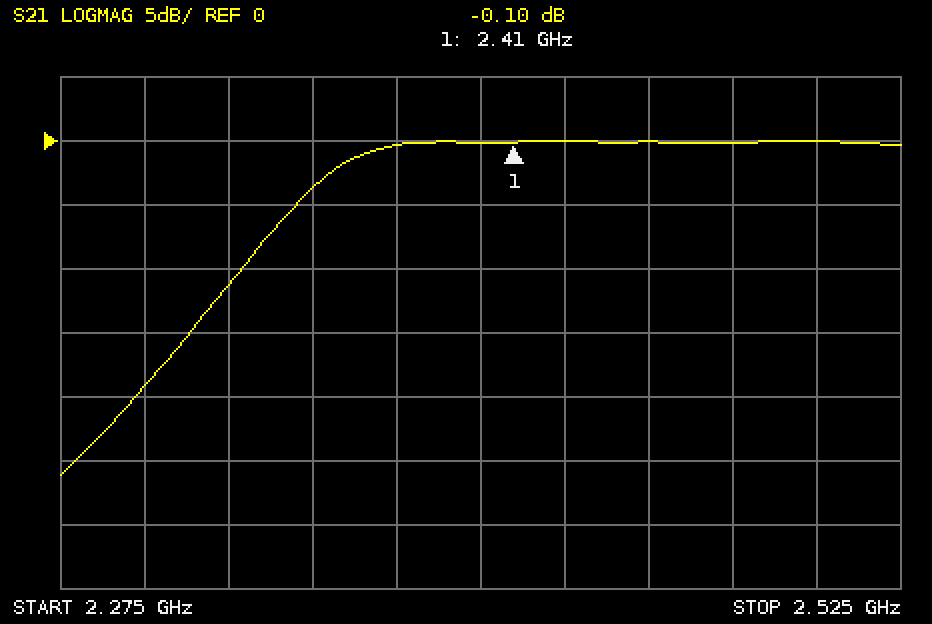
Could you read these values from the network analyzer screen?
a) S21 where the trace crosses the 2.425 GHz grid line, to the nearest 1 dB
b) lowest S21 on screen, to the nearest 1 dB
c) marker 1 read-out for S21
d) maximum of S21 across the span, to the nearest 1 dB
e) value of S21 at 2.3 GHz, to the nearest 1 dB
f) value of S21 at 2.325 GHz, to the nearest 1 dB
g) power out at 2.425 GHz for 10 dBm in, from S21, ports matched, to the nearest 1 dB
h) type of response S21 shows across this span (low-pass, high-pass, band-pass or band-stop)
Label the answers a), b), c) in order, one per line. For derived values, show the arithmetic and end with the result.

a) 0 dB
b) -26 dB
c) -0.10 dB
d) 0 dB
e) -19 dB
f) -11 dB
g) 10 dBm + (0 dB) = 10 dBm
h) high-pass
